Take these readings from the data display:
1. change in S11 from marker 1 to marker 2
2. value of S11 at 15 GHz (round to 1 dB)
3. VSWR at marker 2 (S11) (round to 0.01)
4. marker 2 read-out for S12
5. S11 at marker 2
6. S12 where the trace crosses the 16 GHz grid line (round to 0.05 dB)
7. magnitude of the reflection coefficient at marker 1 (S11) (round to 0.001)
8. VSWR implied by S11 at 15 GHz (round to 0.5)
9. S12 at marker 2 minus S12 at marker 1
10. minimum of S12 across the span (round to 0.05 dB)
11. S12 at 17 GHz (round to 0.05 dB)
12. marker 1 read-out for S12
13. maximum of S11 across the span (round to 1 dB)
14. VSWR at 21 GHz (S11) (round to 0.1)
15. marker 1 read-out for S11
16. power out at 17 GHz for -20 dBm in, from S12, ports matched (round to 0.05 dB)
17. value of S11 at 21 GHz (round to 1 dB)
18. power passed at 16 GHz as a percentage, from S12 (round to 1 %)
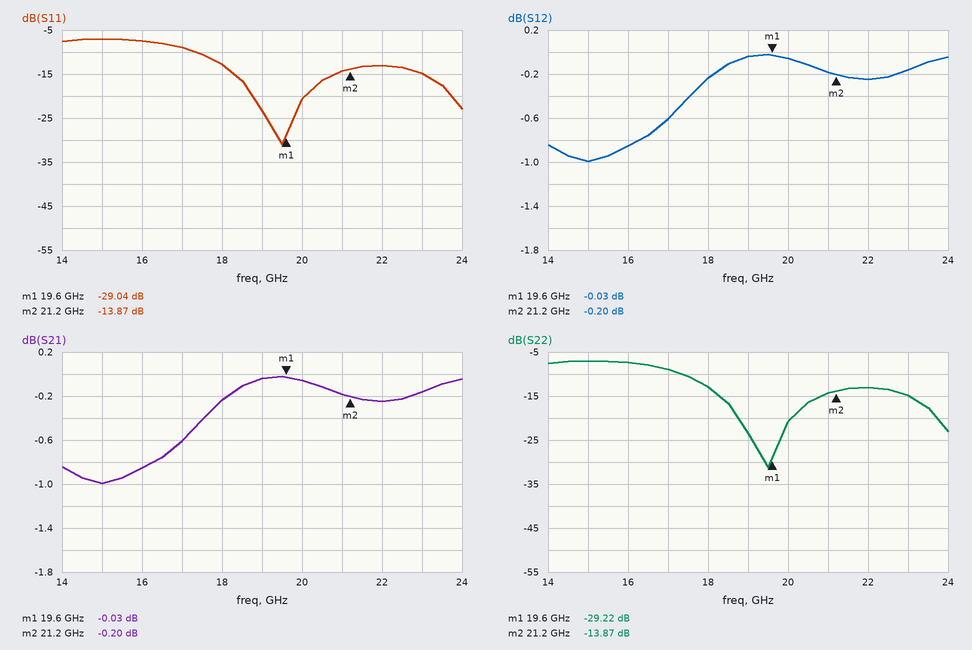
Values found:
15.17 dB
-7 dB
1.51
-0.20 dB
-13.87 dB
-0.85 dB
0.035
2.5
-0.17 dB
-1.00 dB
-0.60 dB
-0.03 dB
-7 dB
1.5
-29.04 dB
-20.60 dBm
-14 dB
82 %
